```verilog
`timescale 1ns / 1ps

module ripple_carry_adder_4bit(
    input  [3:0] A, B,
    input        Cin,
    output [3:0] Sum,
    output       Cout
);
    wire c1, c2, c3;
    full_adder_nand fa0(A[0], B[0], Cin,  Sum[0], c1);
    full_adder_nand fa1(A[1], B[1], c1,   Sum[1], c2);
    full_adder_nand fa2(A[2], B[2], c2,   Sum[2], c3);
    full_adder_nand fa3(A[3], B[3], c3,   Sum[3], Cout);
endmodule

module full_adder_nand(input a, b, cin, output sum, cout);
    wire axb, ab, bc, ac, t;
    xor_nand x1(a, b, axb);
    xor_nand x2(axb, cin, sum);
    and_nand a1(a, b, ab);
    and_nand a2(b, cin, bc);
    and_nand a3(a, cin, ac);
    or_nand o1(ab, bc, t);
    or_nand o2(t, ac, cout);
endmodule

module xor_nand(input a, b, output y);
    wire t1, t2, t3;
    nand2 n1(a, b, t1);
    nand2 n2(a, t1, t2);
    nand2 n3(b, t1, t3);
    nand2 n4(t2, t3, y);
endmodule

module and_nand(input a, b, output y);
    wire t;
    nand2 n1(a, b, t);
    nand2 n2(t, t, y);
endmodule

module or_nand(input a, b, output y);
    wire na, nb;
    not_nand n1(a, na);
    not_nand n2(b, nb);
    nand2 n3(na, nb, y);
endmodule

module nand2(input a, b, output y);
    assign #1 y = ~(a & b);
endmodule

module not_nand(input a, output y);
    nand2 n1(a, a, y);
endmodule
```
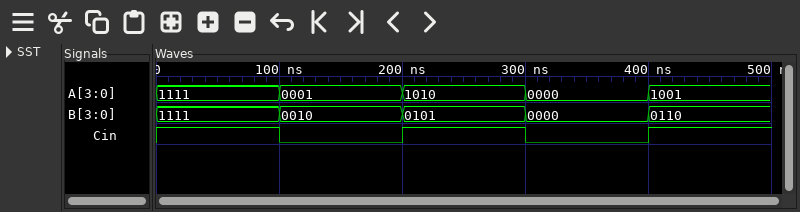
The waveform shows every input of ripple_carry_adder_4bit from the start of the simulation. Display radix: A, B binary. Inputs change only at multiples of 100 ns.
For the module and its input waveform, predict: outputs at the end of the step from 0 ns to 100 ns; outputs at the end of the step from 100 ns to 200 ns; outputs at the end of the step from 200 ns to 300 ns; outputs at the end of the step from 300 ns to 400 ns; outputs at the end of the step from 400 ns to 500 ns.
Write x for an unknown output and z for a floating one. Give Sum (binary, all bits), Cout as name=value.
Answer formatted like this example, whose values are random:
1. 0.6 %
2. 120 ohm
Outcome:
1. Sum=1111, Cout=1
2. Sum=0011, Cout=0
3. Sum=0000, Cout=1
4. Sum=0000, Cout=0
5. Sum=0000, Cout=1
